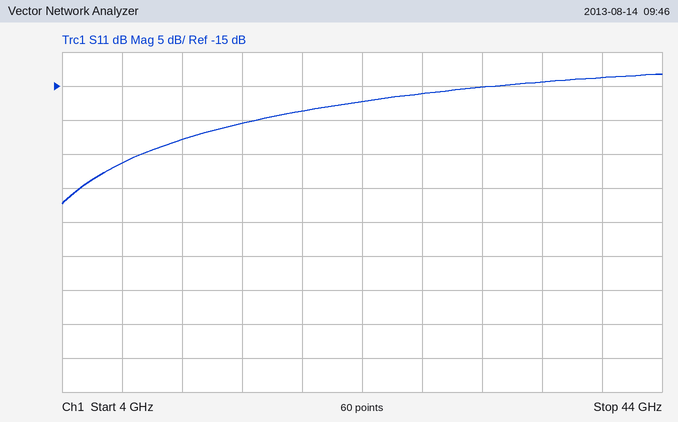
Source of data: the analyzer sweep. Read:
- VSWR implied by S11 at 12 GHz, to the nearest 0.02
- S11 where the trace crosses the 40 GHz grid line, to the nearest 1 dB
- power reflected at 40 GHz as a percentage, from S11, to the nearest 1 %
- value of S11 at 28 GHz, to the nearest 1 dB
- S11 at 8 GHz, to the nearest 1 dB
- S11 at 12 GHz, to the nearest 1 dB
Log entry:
1.16
-14 dB
4 %
-16 dB
-26 dB
-23 dB
